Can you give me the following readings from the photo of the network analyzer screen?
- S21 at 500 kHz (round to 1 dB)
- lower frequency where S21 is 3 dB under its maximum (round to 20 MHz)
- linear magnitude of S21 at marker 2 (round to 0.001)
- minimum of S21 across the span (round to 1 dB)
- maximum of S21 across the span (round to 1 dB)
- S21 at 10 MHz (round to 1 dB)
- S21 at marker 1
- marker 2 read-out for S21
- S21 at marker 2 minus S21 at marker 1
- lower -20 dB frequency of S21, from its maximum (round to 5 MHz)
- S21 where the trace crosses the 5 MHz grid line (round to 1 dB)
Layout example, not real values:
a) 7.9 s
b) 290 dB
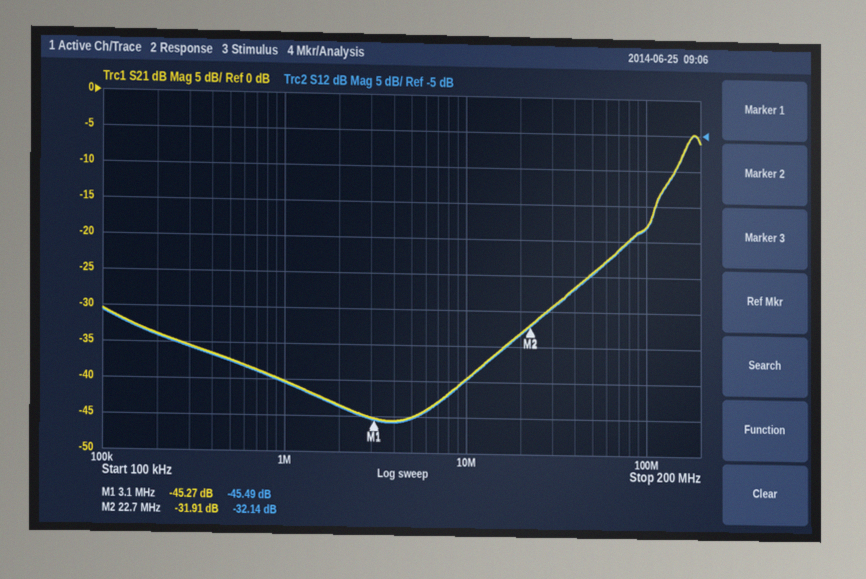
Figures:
a) -37 dB
b) 160 MHz
c) 0.025
d) -46 dB
e) -5 dB
f) -40 dB
g) -45.27 dB
h) -31.91 dB
i) 13.36 dB
j) 50 MHz
k) -45 dB
